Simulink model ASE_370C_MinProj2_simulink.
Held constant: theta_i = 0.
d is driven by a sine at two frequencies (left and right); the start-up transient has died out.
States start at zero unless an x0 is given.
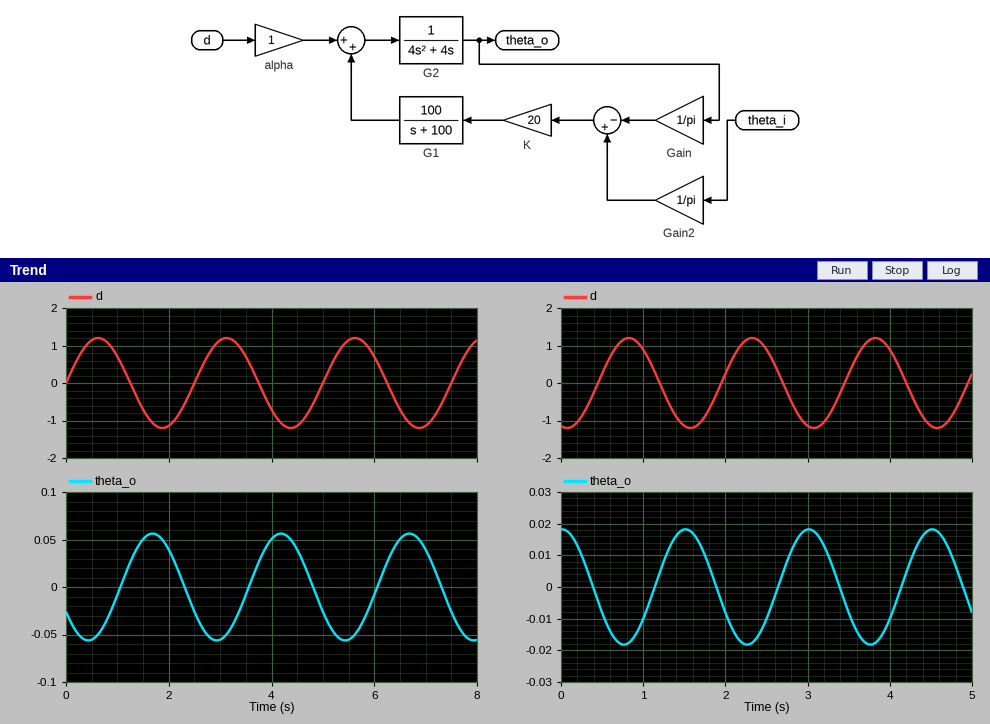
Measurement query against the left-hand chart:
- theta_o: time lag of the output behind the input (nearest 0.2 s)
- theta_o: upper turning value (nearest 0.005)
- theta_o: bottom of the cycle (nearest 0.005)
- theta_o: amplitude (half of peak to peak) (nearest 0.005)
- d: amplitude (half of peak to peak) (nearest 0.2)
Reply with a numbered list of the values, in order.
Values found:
1. 1.0 s
2. 0.055
3. -0.055
4. 0.055
5. 1.2
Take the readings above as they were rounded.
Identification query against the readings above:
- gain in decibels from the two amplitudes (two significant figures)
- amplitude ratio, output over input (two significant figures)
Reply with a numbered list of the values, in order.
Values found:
1. -27 dB
2. 0.046
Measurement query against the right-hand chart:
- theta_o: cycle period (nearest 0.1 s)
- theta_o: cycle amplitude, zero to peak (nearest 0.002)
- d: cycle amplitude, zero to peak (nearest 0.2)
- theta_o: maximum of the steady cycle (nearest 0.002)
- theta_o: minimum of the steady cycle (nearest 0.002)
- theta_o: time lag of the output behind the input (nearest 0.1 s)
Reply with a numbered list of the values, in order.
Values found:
1. 1.5 s
2. 0.018
3. 1.2
4. 0.018
5. -0.018
6. 0.7 s
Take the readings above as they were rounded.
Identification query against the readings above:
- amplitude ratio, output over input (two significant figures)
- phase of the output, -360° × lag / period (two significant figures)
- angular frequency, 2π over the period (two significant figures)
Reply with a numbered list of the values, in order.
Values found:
1. 0.015
2. -170°
3. 4.2 rad/s
